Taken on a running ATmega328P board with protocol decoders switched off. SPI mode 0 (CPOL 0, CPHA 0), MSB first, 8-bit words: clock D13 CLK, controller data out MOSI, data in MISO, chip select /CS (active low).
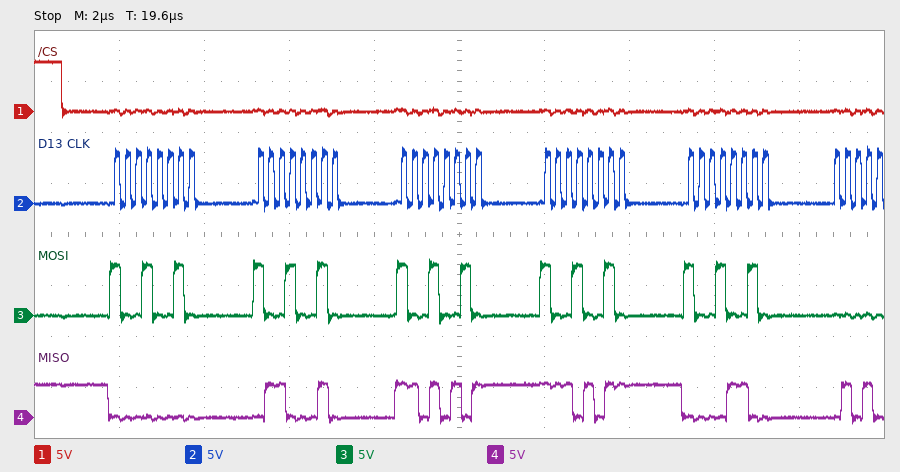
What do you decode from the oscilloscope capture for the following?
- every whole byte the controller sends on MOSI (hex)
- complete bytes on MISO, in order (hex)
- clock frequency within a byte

92 92 92 92 92
00 62 D5 EB 0C
4 MHz
